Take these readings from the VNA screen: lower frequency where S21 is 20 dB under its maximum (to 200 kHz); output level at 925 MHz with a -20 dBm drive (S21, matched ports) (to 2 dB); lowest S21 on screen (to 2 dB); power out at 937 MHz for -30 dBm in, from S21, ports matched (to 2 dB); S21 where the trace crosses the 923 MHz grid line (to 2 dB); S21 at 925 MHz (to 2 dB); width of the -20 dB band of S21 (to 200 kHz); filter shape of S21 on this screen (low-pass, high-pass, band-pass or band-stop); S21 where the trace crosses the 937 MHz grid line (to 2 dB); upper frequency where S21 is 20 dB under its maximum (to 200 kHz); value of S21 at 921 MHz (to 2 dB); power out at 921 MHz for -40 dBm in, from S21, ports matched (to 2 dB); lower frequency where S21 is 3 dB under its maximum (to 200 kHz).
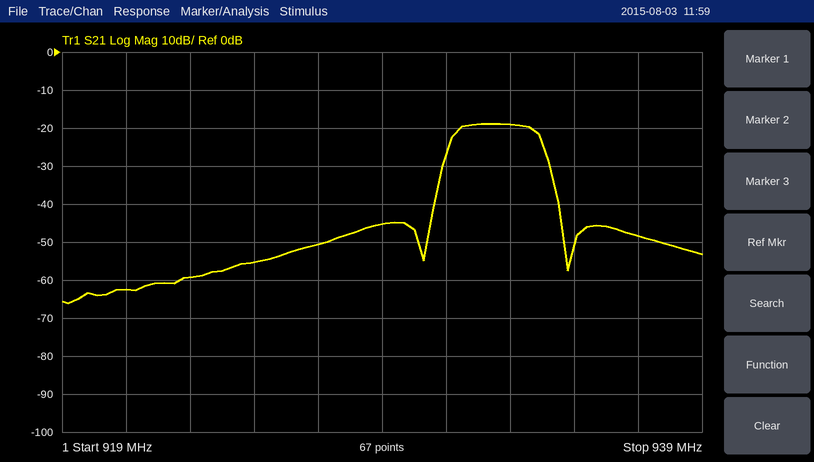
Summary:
930.6 MHz
-76 dBm
-66 dB
-78 dBm
-60 dB
-56 dB
3.8 MHz
band-pass
-48 dB
934.4 MHz
-62 dB
-102 dBm
931.2 MHz
